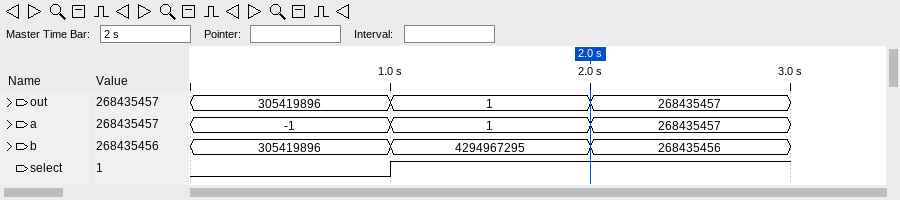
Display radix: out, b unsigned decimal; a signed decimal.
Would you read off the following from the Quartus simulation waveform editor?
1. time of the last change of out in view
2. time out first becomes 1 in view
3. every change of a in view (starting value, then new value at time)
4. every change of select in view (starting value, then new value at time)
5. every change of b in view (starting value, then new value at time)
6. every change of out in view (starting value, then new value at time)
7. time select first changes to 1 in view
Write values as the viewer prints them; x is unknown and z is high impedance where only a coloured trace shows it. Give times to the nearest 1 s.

2 s
1 s
-1, 1 at 1 s, 268435457 at 2 s
0, 1 at 1 s
305419896, 4294967295 at 1 s, 268435456 at 2 s
305419896, 1 at 1 s, 268435457 at 2 s
1 s
